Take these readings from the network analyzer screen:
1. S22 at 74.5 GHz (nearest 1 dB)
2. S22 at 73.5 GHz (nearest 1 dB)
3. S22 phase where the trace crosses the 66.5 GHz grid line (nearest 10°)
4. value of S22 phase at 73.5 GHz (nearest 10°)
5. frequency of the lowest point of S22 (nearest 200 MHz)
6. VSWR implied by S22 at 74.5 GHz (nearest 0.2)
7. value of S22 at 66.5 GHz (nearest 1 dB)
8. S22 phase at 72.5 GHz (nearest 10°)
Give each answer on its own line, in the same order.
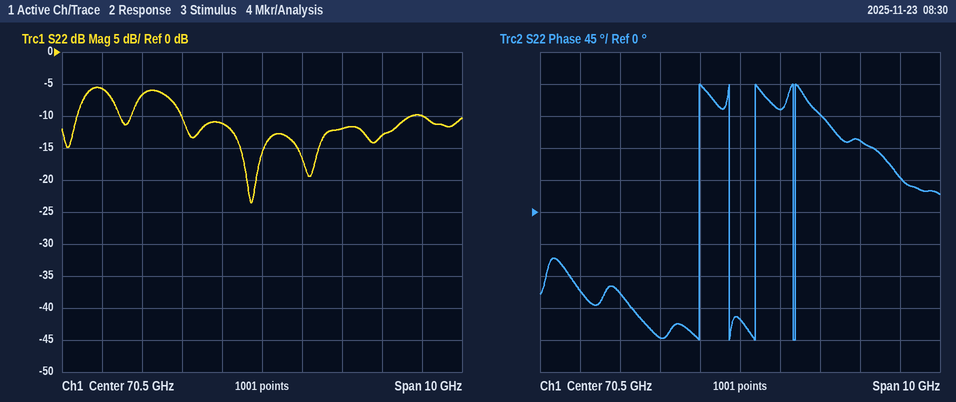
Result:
-10 dB
-13 dB
-110°
100°
70.2 GHz
2.0
-6 dB
140°
